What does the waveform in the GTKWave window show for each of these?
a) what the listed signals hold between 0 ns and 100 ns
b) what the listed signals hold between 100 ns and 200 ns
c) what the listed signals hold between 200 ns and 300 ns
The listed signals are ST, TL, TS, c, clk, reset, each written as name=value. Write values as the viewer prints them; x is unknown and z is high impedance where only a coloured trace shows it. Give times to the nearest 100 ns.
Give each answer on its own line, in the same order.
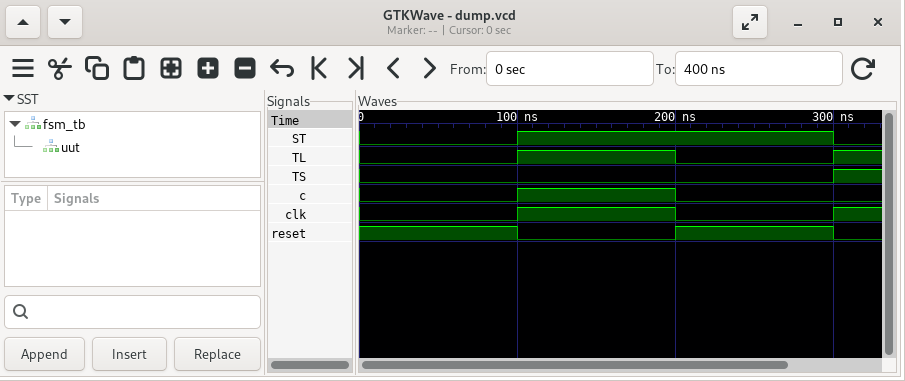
ST=0, TL=0, TS=0, c=0, clk=0, reset=1
ST=1, TL=1, TS=0, c=1, clk=1, reset=0
ST=1, TL=0, TS=0, c=0, clk=0, reset=1
